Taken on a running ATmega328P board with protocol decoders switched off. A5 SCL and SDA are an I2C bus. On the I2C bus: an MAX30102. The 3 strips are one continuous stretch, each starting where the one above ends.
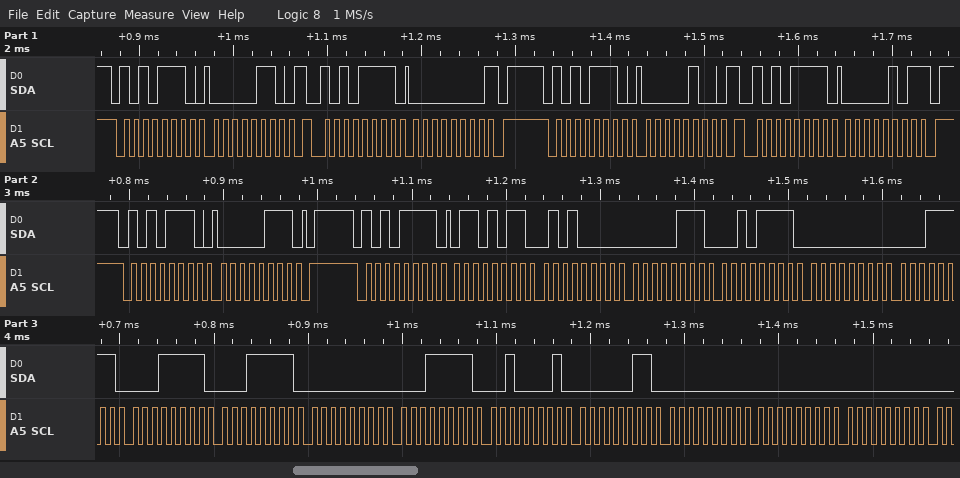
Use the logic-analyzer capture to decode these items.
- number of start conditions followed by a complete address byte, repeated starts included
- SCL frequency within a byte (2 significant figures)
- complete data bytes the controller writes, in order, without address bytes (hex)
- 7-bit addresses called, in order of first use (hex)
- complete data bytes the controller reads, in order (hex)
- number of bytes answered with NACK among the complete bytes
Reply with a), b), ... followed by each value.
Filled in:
a) 6
b) 100 kHz
c) 06 04 07
d) 0x57
e) 00 05 6B 50 07 2F 00 1F 1F 1F 00 1F 21 03 00 00 00
f) 2
